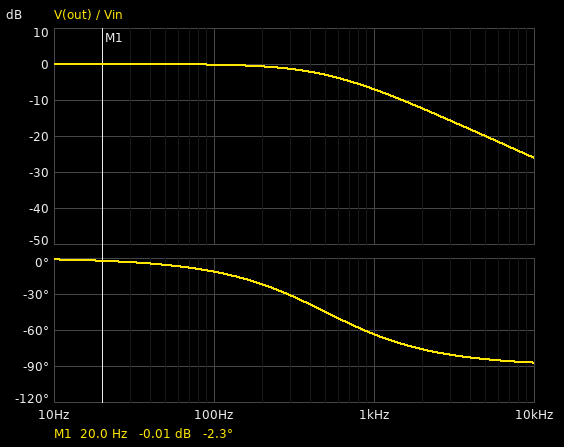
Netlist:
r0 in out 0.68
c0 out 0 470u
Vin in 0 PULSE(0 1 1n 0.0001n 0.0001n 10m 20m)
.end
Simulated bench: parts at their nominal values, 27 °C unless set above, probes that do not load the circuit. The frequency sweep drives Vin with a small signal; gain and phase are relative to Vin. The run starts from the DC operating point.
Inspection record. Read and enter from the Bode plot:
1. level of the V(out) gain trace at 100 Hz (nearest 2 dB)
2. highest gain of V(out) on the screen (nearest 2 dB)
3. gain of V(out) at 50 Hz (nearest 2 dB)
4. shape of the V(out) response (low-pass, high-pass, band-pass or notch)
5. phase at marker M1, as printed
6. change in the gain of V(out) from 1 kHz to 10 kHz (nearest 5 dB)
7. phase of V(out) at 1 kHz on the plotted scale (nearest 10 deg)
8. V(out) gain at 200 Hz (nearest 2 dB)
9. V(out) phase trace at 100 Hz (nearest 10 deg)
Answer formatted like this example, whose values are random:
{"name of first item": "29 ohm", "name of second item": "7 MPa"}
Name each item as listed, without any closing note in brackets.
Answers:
{"level of the V(out) gain trace at 100 Hz": "0 dB", "highest gain of V(out) on the screen": "0 dB", "gain of V(out) at 50 Hz": "0 dB", "shape of the V(out) response": "low-pass", "phase at marker M1, as printed": "-2.3 deg", "change in the gain of V(out) from 1 kHz to 10 kHz": "-20 dB", "phase of V(out) at 1 kHz on the plotted scale": "-60 deg", "V(out) gain at 200 Hz": "0 dB", "V(out) phase trace at 100 Hz": "-10 deg"}
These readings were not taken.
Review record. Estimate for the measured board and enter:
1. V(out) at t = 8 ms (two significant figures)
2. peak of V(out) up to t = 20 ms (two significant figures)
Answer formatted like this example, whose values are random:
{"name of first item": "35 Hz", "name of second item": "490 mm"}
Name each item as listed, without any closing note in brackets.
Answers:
{"V(out) at t = 8 ms": "1.0 V", "peak of V(out) up to t = 20 ms": "1.0 V"}
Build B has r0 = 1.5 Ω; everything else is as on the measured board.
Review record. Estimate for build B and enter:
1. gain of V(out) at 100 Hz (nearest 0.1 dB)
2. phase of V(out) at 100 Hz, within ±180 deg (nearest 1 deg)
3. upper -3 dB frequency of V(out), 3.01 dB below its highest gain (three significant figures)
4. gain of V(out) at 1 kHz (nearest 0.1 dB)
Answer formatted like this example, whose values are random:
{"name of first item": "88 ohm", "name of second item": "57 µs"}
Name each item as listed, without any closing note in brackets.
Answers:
{"gain of V(out) at 100 Hz": "-0.8 dB", "phase of V(out) at 100 Hz, within ±180 deg": "-24 deg", "upper -3 dB frequency of V(out), 3.01 dB below its highest gain": "226 Hz", "gain of V(out) at 1 kHz": "-13.1 dB"}
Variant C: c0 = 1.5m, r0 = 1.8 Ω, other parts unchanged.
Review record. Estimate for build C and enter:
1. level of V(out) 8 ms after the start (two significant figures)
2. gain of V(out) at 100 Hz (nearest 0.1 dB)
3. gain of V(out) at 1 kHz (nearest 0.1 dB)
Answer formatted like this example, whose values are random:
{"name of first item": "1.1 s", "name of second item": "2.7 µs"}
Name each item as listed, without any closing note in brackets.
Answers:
{"level of V(out) 8 ms after the start": "950 mV", "gain of V(out) at 100 Hz": "-5.9 dB", "gain of V(out) at 1 kHz": "-24.6 dB"}
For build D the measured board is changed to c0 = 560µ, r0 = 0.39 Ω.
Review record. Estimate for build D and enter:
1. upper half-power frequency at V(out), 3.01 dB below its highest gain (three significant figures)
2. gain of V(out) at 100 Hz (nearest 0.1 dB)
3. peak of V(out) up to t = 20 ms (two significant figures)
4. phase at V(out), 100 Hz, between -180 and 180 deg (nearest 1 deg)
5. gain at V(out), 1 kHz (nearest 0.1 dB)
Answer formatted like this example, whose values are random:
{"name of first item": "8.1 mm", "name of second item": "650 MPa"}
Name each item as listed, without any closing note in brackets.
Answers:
{"upper half-power frequency at V(out), 3.01 dB below its highest gain": "729 Hz", "gain of V(out) at 100 Hz": "-0.1 dB", "peak of V(out) up to t = 20 ms": "1.0 V", "phase at V(out), 100 Hz, between -180 and 180 deg": "-8 deg", "gain at V(out), 1 kHz": "-4.6 dB"}
